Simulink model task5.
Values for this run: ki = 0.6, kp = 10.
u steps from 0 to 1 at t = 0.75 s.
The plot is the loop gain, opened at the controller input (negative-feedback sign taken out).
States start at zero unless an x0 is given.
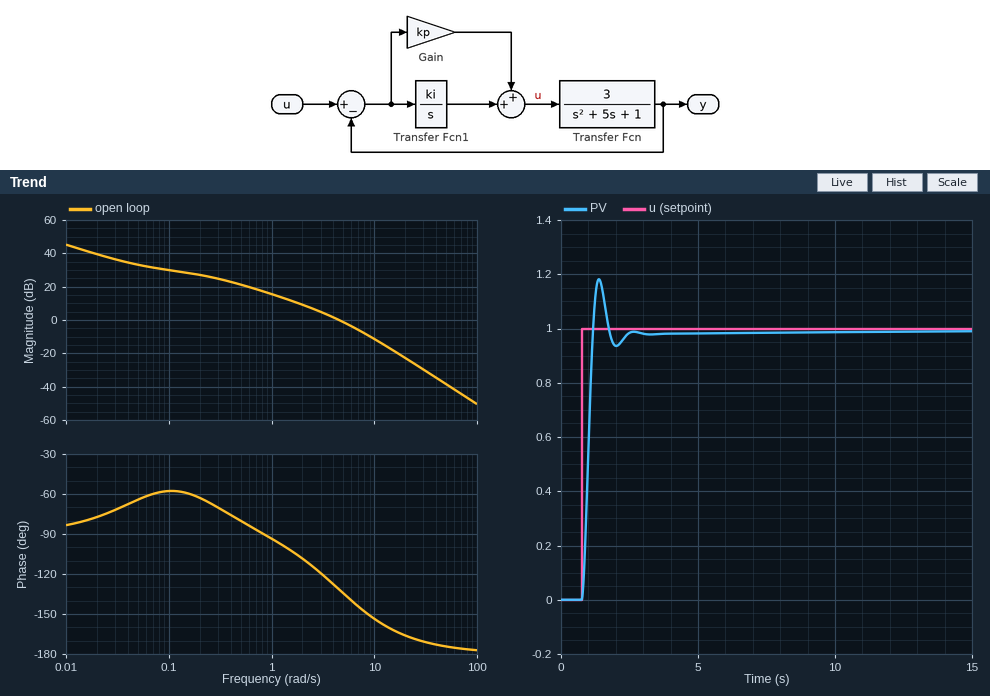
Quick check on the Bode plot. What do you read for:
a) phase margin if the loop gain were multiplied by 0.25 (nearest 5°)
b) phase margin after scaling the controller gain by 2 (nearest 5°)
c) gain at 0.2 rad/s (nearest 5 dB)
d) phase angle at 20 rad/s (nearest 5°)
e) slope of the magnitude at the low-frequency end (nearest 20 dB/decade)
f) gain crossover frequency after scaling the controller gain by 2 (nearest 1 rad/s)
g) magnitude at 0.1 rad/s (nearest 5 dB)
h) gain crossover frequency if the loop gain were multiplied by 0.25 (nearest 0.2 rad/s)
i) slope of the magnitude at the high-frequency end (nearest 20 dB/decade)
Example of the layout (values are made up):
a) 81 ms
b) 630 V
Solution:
a) 80°
b) 35°
c) 25 dB
d) -165°
e) -20 dB/decade
f) 7 rad/s
g) 30 dB
h) 1.4 rad/s
i) -40 dB/decade
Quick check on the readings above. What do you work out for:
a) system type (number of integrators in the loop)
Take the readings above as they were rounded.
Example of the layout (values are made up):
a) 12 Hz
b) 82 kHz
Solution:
a) 1
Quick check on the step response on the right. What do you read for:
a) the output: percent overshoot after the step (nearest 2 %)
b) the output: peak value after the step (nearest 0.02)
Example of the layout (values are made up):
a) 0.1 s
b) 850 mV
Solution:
a) 18 %
b) 1.18
